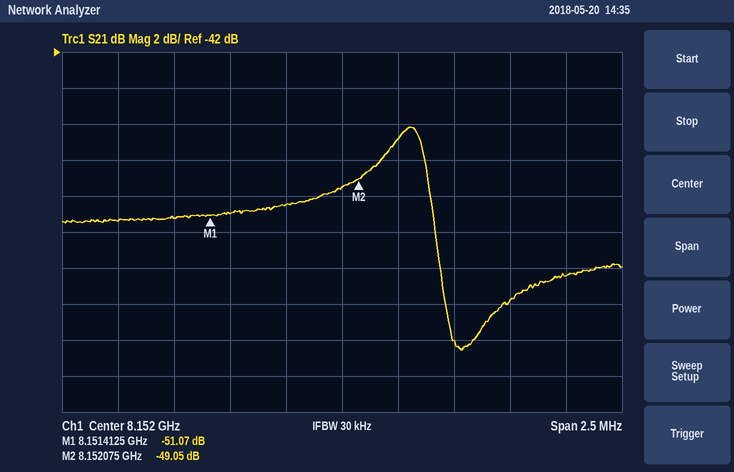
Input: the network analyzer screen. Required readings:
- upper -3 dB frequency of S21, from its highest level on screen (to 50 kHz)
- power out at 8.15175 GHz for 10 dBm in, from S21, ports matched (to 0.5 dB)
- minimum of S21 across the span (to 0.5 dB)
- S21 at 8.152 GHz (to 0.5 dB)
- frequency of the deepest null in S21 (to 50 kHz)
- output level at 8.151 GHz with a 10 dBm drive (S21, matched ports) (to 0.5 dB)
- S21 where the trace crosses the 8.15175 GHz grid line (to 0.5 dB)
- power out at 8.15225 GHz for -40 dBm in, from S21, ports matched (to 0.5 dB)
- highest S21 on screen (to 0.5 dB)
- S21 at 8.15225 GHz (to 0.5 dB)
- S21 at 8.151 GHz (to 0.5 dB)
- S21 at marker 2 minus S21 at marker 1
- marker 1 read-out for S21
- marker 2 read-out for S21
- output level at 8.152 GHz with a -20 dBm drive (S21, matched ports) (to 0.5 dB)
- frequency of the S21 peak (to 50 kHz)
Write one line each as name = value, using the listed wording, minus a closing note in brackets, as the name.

upper -3 dB frequency of S21, from its highest level on screen = 8.15240 GHz
power out at 8.15175 GHz for 10 dBm in, from S21, ports matched = -40.5 dBm
minimum of S21 across the span = -58.5 dB
S21 at 8.152 GHz = -49.5 dB
frequency of the deepest null in S21 = 8.15255 GHz
output level at 8.151 GHz with a 10 dBm drive (S21, matched ports) = -41.5 dBm
S21 where the trace crosses the 8.15175 GHz grid line = -50.5 dB
power out at 8.15225 GHz for -40 dBm in, from S21, ports matched = -87.0 dBm
highest S21 on screen = -46.0 dB
S21 at 8.15225 GHz = -47.0 dB
S21 at 8.151 GHz = -51.5 dB
S21 at marker 2 minus S21 at marker 1 = 2.02 dB
marker 1 read-out for S21 = -51.07 dB
marker 2 read-out for S21 = -49.05 dB
output level at 8.152 GHz with a -20 dBm drive (S21, matched ports) = -69.5 dBm
frequency of the S21 peak = 8.15230 GHz
